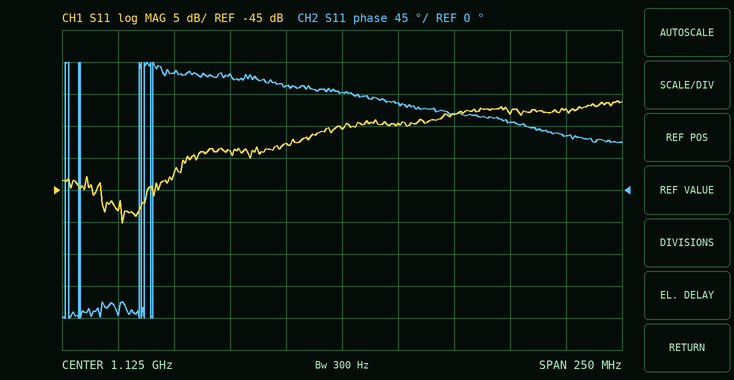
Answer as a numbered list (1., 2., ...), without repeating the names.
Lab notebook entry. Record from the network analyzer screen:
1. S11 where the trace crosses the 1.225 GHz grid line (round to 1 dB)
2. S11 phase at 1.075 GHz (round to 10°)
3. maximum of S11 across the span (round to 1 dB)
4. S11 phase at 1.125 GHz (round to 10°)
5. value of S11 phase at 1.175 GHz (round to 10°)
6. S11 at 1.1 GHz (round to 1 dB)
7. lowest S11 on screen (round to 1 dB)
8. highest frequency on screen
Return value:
1. -32 dB
2. 160°
3. -31 dB
4. 140°
5. 110°
6. -38 dB
7. -50 dB
8. 1.25 GHz
